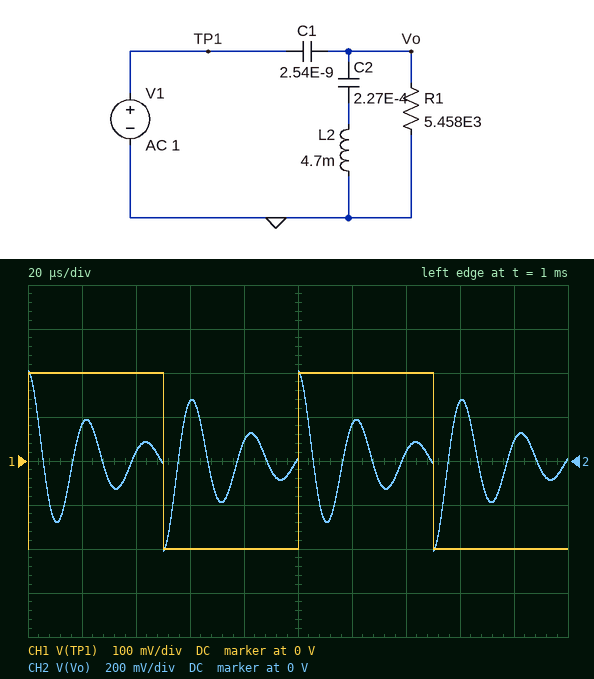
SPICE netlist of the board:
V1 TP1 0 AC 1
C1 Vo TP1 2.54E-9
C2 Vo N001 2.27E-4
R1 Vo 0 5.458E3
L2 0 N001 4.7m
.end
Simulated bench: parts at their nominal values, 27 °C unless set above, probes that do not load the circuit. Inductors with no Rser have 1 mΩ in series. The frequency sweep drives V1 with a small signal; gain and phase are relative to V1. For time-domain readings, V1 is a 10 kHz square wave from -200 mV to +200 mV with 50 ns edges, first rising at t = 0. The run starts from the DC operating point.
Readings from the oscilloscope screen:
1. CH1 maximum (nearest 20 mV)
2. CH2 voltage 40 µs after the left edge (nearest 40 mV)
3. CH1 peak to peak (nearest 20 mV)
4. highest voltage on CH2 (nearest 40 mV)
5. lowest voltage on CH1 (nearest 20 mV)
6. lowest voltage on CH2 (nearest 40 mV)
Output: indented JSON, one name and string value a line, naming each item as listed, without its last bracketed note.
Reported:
{
  "CH1 maximum": "200 mV",
  "CH2 voltage 40 µs after the left edge": "40 mV",
  "CH1 peak to peak": "400 mV",
  "highest voltage on CH2": "400 mV",
  "lowest voltage on CH1": "-200 mV",
  "lowest voltage on CH2": "-400 mV"
}
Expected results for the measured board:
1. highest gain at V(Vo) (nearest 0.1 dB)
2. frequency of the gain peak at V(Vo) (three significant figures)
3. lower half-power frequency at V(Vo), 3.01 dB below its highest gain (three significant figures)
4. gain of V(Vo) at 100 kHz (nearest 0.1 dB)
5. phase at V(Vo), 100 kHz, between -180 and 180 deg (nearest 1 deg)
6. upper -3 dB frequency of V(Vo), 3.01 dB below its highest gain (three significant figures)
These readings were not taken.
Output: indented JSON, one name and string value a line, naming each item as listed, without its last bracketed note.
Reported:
{
  "highest gain at V(Vo)": "12.1 dB",
  "frequency of the gain peak at V(Vo)": "46.8 kHz",
  "lower half-power frequency at V(Vo), 3.01 dB below its highest gain": "41.8 kHz",
  "gain of V(Vo) at 100 kHz": "2.0 dB",
  "phase at V(Vo), 100 kHz, between -180 and 180 deg": "8 deg",
  "upper -3 dB frequency of V(Vo), 3.01 dB below its highest gain": "54.2 kHz"
}
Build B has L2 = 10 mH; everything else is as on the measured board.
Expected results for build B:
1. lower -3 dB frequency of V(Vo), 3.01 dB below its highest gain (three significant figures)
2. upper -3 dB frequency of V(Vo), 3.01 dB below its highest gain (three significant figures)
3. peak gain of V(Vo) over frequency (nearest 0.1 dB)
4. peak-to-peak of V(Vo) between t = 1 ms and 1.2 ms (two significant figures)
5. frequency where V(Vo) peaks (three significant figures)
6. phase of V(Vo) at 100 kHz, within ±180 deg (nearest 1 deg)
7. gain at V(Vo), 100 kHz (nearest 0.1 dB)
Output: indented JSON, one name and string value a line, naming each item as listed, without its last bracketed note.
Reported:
{
  "lower -3 dB frequency of V(Vo), 3.01 dB below its highest gain": "27.8 kHz",
  "upper -3 dB frequency of V(Vo), 3.01 dB below its highest gain": "41.6 kHz",
  "peak gain of V(Vo) over frequency": "8.9 dB",
  "peak-to-peak of V(Vo) between t = 1 ms and 1.2 ms": "930 mV",
  "frequency where V(Vo) peaks": "32.7 kHz",
  "phase of V(Vo) at 100 kHz, within ±180 deg": "7 deg",
  "gain at V(Vo), 100 kHz": "0.8 dB"
}
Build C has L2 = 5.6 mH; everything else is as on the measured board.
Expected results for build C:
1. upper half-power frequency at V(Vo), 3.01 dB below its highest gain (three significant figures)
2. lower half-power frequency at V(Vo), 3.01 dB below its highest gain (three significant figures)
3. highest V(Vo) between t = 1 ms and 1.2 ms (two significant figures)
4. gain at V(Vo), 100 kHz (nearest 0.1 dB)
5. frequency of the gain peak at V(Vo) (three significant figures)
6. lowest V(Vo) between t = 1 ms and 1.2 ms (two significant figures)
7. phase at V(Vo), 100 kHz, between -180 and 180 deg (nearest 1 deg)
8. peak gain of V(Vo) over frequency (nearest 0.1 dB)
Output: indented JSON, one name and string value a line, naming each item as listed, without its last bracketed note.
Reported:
{
  "upper half-power frequency at V(Vo), 3.01 dB below its highest gain": "50.7 kHz",
  "lower half-power frequency at V(Vo), 3.01 dB below its highest gain": "38.0 kHz",
  "highest V(Vo) between t = 1 ms and 1.2 ms": "350 mV",
  "gain at V(Vo), 100 kHz": "1.6 dB",
  "frequency of the gain peak at V(Vo)": "43.0 kHz",
  "lowest V(Vo) between t = 1 ms and 1.2 ms": "-350 mV",
  "phase at V(Vo), 100 kHz, between -180 and 180 deg": "8 deg",
  "peak gain of V(Vo) over frequency": "11.4 dB"
}
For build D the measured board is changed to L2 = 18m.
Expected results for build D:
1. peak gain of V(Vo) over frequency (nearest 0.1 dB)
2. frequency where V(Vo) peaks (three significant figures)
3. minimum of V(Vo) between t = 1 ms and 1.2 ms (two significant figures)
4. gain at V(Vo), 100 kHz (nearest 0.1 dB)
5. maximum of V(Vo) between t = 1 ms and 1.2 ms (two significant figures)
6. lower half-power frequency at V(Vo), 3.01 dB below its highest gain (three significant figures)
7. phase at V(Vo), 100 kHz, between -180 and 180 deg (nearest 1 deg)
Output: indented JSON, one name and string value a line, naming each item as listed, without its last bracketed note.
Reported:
{
  "peak gain of V(Vo) over frequency": "6.5 dB",
  "frequency where V(Vo) peaks": "25.1 kHz",
  "minimum of V(Vo) between t = 1 ms and 1.2 ms": "-370 mV",
  "gain at V(Vo), 100 kHz": "0.4 dB",
  "maximum of V(Vo) between t = 1 ms and 1.2 ms": "370 mV",
  "lower half-power frequency at V(Vo), 3.01 dB below its highest gain": "20.2 kHz",
  "phase at V(Vo), 100 kHz, between -180 and 180 deg": "7 deg"
}
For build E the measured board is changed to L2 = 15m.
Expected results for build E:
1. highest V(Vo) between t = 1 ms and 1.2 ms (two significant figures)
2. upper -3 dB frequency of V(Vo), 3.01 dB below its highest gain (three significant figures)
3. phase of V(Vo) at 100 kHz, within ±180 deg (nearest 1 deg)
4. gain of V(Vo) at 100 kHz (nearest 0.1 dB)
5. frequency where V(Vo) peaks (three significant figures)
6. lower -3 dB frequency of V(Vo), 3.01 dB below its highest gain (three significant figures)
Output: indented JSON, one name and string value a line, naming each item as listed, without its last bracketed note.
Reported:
{
  "highest V(Vo) between t = 1 ms and 1.2 ms": "410 mV",
  "upper -3 dB frequency of V(Vo), 3.01 dB below its highest gain": "37.7 kHz",
  "phase of V(Vo) at 100 kHz, within ±180 deg": "7 deg",
  "gain of V(Vo) at 100 kHz": "0.5 dB",
  "frequency where V(Vo) peaks": "27.2 kHz",
  "lower -3 dB frequency of V(Vo), 3.01 dB below its highest gain": "22.3 kHz"
}
